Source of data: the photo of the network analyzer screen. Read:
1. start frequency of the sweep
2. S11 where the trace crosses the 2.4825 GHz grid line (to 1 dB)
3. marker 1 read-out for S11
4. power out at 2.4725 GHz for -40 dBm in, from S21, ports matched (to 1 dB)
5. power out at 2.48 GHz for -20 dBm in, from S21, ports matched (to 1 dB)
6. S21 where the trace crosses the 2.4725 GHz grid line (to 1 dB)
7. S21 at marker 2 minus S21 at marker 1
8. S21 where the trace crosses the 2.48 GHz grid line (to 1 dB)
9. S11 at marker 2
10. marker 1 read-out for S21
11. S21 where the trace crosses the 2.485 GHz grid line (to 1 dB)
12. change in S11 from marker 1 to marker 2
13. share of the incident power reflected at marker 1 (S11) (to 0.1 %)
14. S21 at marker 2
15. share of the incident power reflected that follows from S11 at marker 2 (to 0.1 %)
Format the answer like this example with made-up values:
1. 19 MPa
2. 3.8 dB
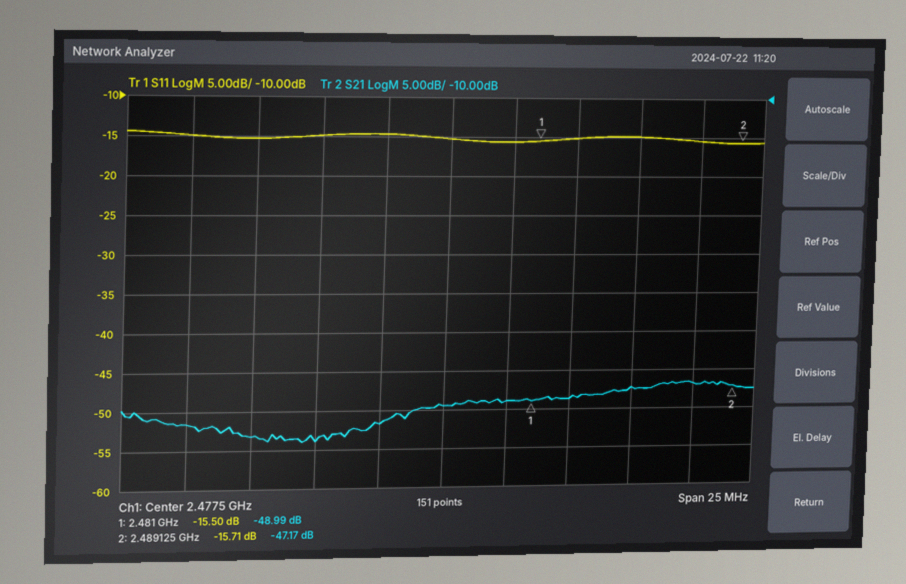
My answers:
1. 2.465 GHz
2. -15 dB
3. -15.50 dB
4. -94 dBm
5. -69 dBm
6. -54 dB
7. 1.82 dB
8. -49 dB
9. -15.71 dB
10. -48.99 dB
11. -47 dB
12. -0.21 dB
13. 2.8 %
14. -47.17 dB
15. 2.7 %
